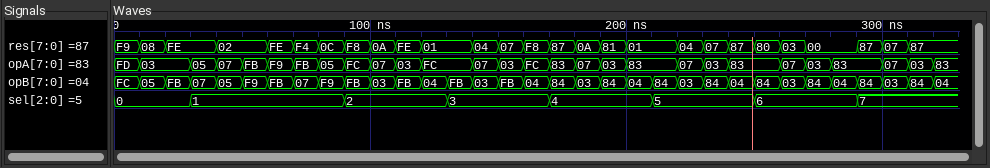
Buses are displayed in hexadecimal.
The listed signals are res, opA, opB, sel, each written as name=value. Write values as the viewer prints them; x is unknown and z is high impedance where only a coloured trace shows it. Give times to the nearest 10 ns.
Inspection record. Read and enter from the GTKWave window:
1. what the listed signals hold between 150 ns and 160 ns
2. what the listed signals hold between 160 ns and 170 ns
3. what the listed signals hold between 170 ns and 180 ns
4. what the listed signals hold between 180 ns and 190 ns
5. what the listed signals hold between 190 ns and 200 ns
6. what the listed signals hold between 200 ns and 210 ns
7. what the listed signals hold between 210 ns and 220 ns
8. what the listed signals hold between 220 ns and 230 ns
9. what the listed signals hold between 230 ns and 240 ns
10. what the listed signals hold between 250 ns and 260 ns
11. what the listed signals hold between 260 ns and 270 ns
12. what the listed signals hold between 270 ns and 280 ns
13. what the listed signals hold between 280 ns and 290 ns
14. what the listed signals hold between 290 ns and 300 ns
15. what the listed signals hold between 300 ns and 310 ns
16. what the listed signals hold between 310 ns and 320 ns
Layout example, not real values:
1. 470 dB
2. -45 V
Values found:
1. res=07, opA=03, opB=FB, sel=3
2. res=F8, opA=FC, opB=04, sel=3
3. res=87, opA=83, opB=84, sel=4
4. res=0A, opA=07, opB=03, sel=4
5. res=81, opA=03, opB=84, sel=4
6. res=01, opA=83, opB=04, sel=4
7. res=01, opA=83, opB=84, sel=5
8. res=04, opA=07, opB=03, sel=5
9. res=07, opA=03, opB=84, sel=5
10. res=80, opA=83, opB=84, sel=6
11. res=03, opA=07, opB=03, sel=6
12. res=00, opA=03, opB=84, sel=6
13. res=00, opA=83, opB=04, sel=6
14. res=87, opA=83, opB=84, sel=7
15. res=07, opA=07, opB=03, sel=7
16. res=87, opA=03, opB=84, sel=7
